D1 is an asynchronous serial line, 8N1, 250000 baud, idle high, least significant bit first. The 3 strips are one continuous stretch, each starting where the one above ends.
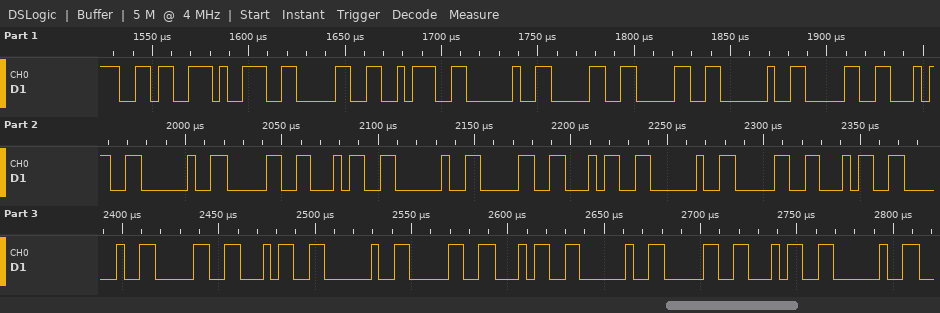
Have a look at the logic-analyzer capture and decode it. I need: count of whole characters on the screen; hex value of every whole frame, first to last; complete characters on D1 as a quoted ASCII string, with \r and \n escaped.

29
36 39 30 3A 20 30 30 20 30 34 20 30 34 20 30 34 20 30 34 20 30 34 20 30 34 20 30 34 20
"690: 00 04 04 04 04 04 04 04 "
